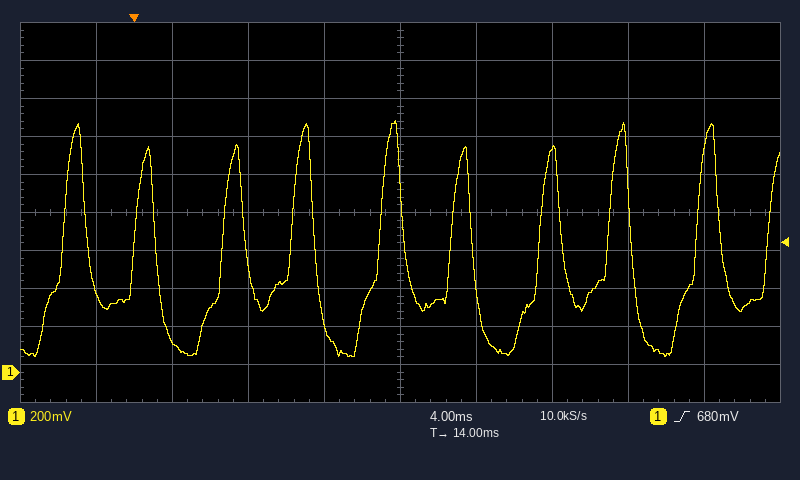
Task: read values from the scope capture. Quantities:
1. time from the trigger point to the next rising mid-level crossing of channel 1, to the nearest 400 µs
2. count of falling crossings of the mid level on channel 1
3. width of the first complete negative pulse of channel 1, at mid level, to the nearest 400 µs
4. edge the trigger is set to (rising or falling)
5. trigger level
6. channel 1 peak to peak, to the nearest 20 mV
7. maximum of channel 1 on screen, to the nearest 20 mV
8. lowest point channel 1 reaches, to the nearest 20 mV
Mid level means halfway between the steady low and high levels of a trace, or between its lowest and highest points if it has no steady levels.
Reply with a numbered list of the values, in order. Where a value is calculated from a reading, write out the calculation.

1. 4.8 ms
2. 9
3. 2.4 ms
4. rising
5. 680 mV
6. 1.32 V − (80 mV) = 1.24 V
7. 1.32 V
8. 80 mV
